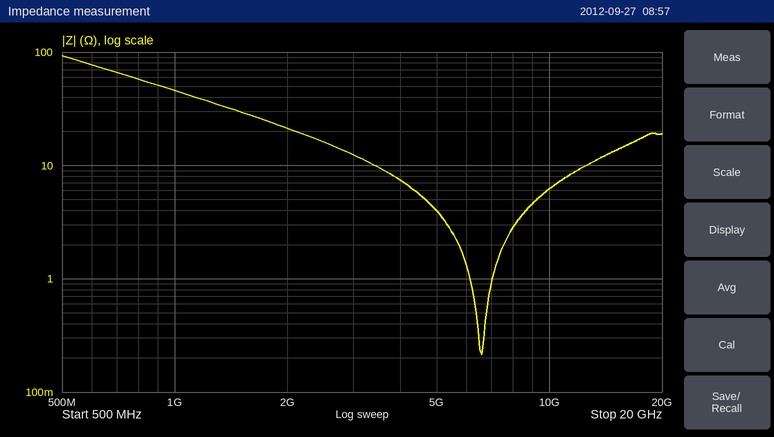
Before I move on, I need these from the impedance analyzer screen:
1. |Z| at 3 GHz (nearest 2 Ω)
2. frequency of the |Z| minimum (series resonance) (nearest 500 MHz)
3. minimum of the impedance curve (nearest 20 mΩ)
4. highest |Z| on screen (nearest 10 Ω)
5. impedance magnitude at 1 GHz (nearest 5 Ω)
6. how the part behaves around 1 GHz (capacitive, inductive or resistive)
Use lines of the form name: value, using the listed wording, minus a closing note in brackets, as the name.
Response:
|Z| at 3 GHz: 12 Ω
frequency of the |Z| minimum (series resonance): 6.5 GHz
minimum of the impedance curve: 220 mΩ
highest |Z| on screen: 90 Ω
impedance magnitude at 1 GHz: 45 Ω
how the part behaves around 1 GHz: capacitive
